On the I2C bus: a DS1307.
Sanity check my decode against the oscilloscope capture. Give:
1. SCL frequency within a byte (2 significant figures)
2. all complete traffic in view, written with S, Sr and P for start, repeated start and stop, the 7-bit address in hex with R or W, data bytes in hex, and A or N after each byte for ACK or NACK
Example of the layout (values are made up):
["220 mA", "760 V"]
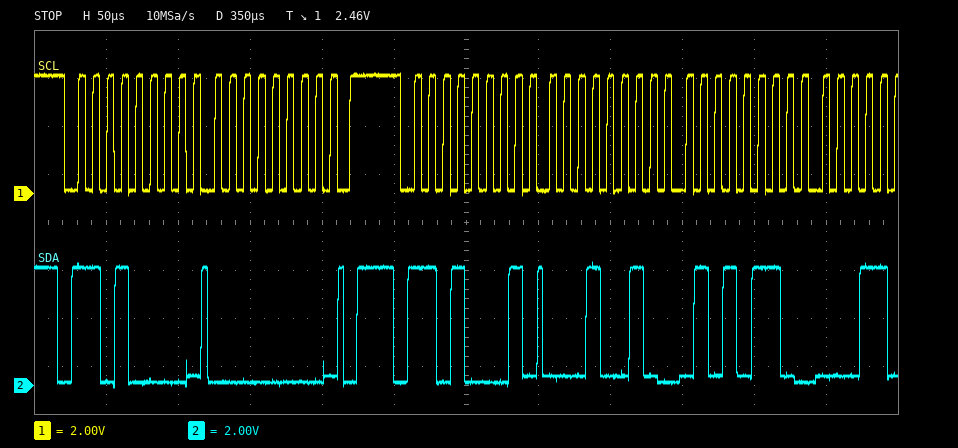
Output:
["100 kHz", "S 68W A 00 A P S 68R A 12 A 56 A"]
